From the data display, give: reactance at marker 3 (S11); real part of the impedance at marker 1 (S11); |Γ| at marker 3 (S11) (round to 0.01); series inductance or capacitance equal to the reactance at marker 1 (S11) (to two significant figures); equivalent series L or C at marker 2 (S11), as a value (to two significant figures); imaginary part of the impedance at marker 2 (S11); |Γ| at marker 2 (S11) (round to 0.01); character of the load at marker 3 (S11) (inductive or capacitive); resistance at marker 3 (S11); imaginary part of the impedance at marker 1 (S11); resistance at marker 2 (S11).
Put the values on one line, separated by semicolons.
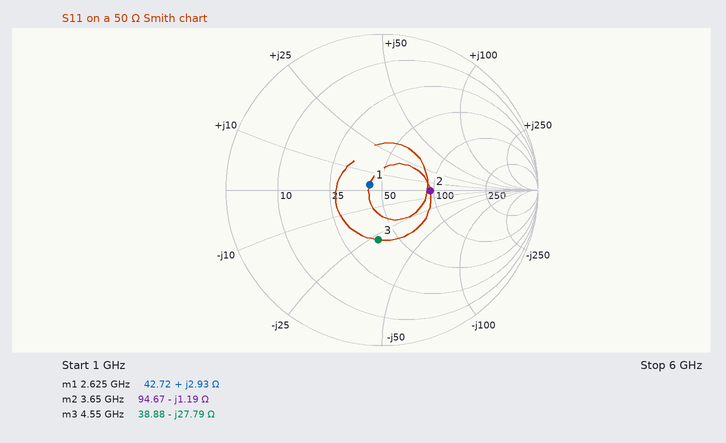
-27.79 Ω; 42.72 Ω; 0.32; 180 pH; 37 pF; -1.19 Ω; 0.31; capacitive; 38.88 Ω; +2.93 Ω; 94.67 Ω
